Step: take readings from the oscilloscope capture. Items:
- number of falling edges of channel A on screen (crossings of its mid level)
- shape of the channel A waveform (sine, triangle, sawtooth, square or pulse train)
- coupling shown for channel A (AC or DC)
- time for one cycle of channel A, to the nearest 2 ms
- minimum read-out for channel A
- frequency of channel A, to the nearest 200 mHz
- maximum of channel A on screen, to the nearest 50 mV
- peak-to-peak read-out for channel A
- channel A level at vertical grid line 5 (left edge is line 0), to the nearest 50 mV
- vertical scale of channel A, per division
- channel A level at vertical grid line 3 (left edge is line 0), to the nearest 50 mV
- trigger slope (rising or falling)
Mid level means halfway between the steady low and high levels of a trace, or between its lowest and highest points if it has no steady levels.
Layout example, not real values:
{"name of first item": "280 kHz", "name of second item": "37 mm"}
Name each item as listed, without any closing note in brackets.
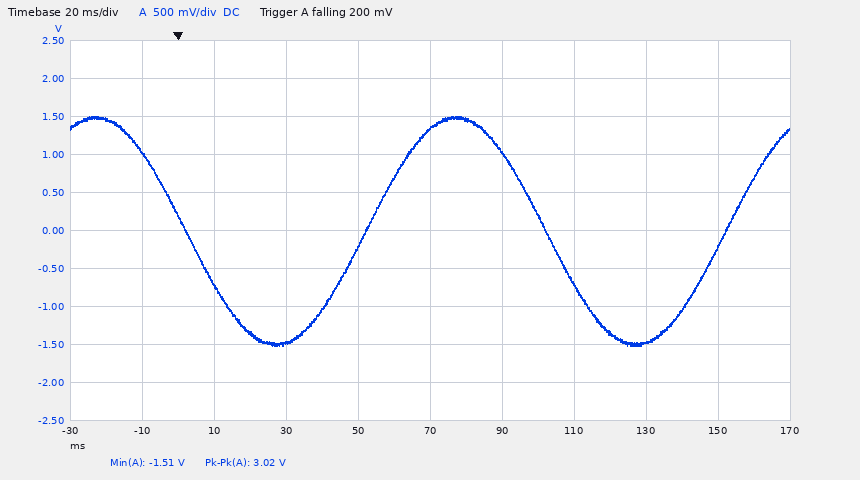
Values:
{"number of falling edges of channel A on screen": "2", "shape of the channel A waveform": "sine", "coupling shown for channel A": "DC", "time for one cycle of channel A, to the nearest 2 ms": "100 ms", "minimum read-out for channel A": "-1.51 V", "frequency of channel A, to the nearest 200 mHz": "10.0 Hz", "maximum of channel A on screen, to the nearest 50 mV": "1.50 V", "peak-to-peak read-out for channel A": "3.02 V", "channel A level at vertical grid line 5 (left edge is line 0), to the nearest 50 mV": "1.35 V", "vertical scale of channel A, per division": "500 mV", "channel A level at vertical grid line 3 (left edge is line 0), to the nearest 50 mV": "-1.50 V", "trigger slope": "falling"}
